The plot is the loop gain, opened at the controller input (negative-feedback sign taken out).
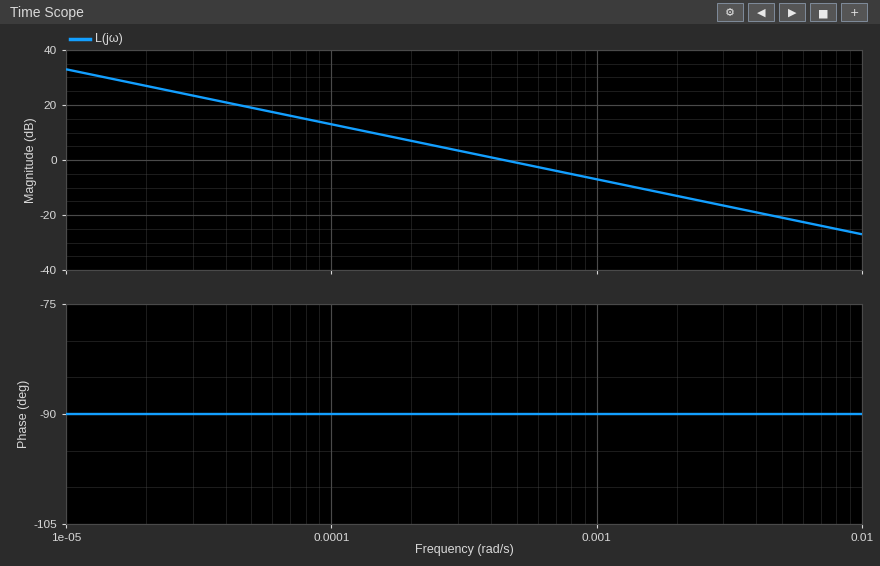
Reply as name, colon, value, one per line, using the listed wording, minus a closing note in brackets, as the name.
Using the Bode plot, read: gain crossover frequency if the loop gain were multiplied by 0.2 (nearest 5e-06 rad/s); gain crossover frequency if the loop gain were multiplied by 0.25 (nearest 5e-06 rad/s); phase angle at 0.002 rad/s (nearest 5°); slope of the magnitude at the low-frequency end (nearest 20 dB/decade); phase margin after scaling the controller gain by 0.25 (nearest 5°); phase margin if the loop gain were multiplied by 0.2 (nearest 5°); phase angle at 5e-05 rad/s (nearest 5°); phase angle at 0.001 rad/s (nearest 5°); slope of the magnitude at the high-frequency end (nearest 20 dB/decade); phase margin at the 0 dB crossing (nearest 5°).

gain crossover frequency if the loop gain were multiplied by 0.2: 0.000090 rad/s
gain crossover frequency if the loop gain were multiplied by 0.25: 0.000110 rad/s
phase angle at 0.002 rad/s: -90°
slope of the magnitude at the low-frequency end: -20 dB/decade
phase margin after scaling the controller gain by 0.25: 90°
phase margin if the loop gain were multiplied by 0.2: 90°
phase angle at 5e-05 rad/s: -90°
phase angle at 0.001 rad/s: -90°
slope of the magnitude at the high-frequency end: -20 dB/decade
phase margin at the 0 dB crossing: 90°
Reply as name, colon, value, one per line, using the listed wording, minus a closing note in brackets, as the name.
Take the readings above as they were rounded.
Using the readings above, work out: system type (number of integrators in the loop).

system type: 1
